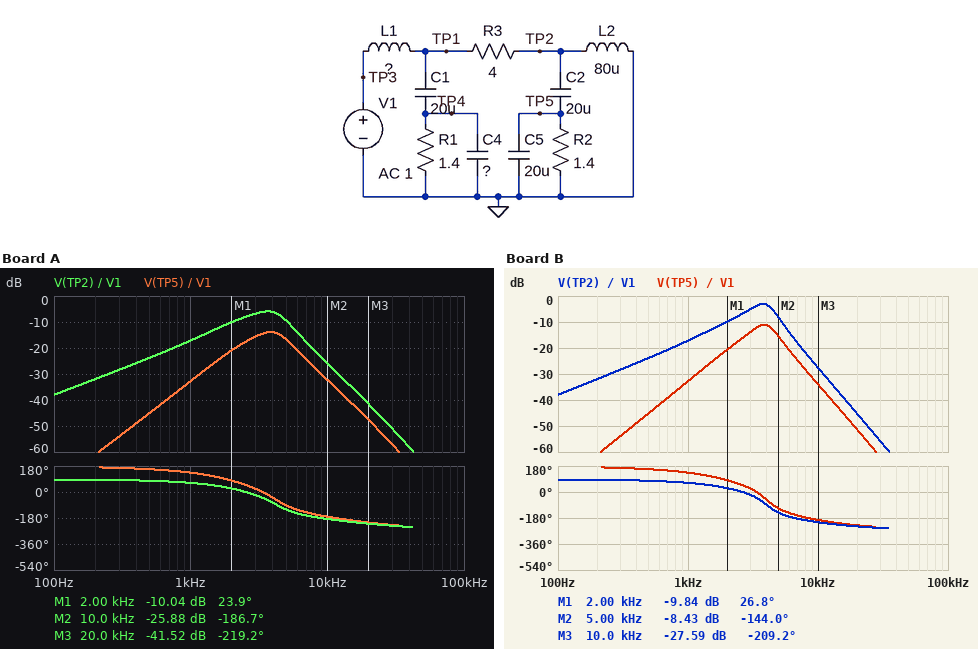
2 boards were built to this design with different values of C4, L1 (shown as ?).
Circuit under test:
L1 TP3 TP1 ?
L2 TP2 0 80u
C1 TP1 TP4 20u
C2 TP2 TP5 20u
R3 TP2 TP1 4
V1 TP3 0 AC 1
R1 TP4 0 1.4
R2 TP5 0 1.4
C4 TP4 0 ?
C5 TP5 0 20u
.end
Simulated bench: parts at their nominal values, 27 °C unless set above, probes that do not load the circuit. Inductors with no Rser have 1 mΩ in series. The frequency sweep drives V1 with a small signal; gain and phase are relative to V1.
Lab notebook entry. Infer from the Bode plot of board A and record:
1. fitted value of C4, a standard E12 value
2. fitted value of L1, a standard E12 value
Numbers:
10 µF
180 µH
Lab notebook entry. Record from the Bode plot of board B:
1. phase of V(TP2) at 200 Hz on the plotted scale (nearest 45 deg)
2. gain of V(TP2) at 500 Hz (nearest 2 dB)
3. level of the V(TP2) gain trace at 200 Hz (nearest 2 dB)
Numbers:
90 deg
-24 dB
-32 dB
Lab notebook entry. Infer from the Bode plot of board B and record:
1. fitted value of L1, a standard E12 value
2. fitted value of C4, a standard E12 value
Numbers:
180 µH
33 µF
